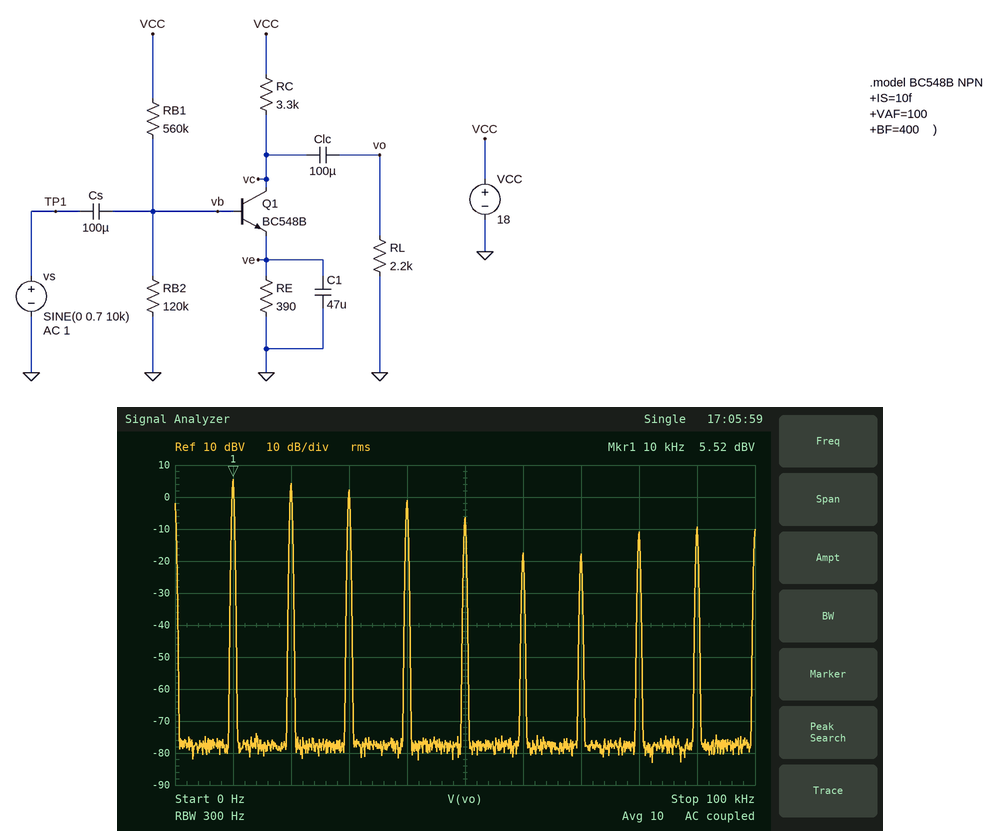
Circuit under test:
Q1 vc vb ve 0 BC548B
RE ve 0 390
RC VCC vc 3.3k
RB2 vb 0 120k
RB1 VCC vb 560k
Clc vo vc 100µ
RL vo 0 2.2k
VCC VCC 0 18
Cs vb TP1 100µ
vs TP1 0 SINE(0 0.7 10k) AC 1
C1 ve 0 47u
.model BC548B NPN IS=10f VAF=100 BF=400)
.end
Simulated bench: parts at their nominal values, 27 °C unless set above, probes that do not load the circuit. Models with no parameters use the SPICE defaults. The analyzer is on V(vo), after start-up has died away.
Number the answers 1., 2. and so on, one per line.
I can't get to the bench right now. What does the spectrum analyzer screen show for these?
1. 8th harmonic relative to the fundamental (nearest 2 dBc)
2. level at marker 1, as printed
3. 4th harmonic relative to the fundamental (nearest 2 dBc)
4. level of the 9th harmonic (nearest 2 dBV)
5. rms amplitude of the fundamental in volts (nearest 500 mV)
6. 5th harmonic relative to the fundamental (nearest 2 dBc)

1. -16 dBc
2. 5.52 dBV
3. -6 dBc
4. -10 dBV
5. 2.0 V
6. -12 dBc
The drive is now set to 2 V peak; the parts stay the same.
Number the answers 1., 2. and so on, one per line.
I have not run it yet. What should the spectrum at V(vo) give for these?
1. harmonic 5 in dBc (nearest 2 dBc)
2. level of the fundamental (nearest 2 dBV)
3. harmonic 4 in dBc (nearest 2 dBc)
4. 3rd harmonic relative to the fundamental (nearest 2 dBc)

1. -4 dBc
2. 2 dBV
3. -2 dBc
4. -2 dBc
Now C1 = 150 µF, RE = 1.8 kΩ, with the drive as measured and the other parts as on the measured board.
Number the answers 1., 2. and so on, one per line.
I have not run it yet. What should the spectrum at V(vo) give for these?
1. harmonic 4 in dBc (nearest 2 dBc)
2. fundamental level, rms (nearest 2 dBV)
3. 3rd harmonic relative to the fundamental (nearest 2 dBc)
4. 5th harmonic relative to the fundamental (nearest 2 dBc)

1. -4 dBc
2. 6 dBV
3. -2 dBc
4. -6 dBc
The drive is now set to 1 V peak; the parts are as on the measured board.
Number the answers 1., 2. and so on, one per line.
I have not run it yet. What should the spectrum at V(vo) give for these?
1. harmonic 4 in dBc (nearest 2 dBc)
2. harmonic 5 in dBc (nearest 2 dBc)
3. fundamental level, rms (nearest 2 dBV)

1. -4 dBc
2. -8 dBc
3. 4 dBV
